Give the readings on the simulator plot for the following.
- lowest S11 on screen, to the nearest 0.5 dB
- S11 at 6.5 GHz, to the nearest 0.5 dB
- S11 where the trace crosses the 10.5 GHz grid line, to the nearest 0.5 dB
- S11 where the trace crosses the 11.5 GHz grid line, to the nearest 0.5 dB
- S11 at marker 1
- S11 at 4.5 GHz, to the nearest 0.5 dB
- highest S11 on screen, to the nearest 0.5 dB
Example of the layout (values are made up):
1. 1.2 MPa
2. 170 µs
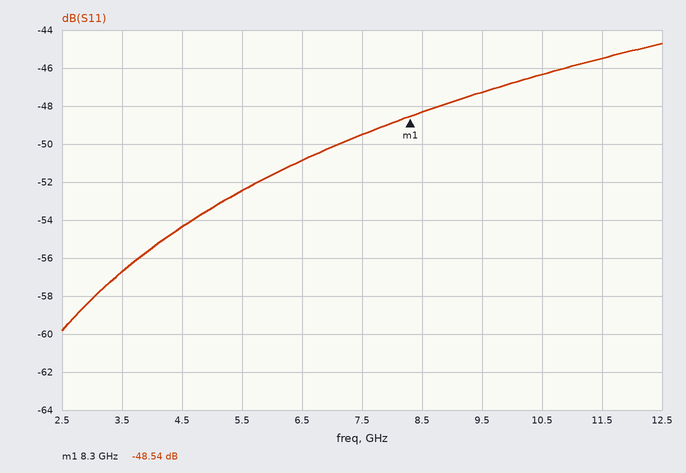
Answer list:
1. -60.0 dB
2. -51.0 dB
3. -46.5 dB
4. -45.5 dB
5. -48.54 dB
6. -54.5 dB
7. -44.5 dB
